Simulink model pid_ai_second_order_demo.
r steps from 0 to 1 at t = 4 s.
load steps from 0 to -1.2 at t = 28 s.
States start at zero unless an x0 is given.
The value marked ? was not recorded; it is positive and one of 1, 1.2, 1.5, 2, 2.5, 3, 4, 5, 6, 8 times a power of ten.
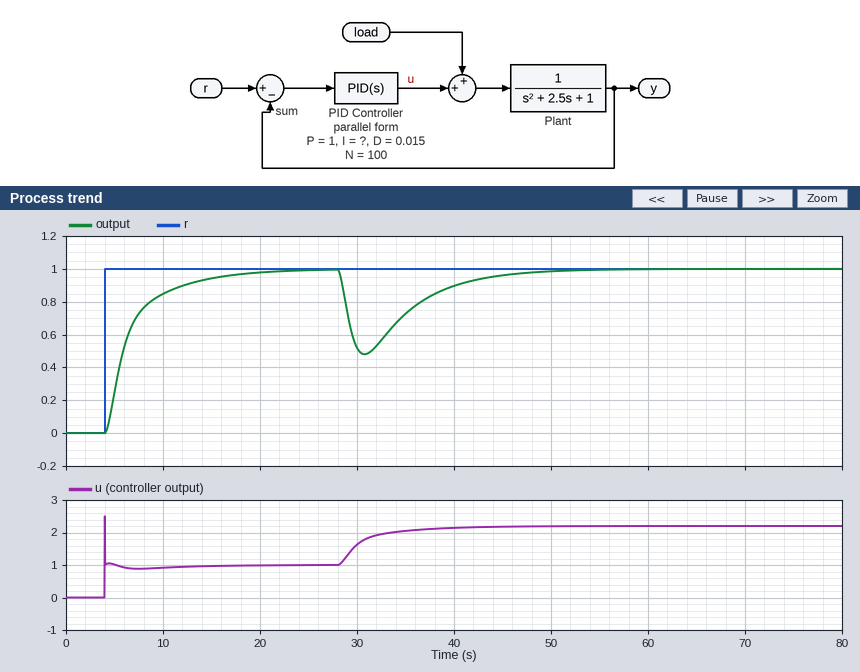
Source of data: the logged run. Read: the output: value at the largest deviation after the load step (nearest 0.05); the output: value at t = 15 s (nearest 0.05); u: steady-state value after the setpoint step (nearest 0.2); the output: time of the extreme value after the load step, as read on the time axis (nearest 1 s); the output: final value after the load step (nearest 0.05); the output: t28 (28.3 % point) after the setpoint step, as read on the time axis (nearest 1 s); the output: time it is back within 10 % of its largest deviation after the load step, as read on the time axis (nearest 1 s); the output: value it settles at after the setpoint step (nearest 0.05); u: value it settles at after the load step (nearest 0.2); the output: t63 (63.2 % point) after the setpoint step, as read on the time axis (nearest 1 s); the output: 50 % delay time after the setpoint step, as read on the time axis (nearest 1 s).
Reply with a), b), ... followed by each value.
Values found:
a) 0.50
b) 0.95
c) 1.0
d) 31 s
e) 1.00
f) 5 s
g) 44 s
h) 1.00
i) 2.2
j) 7 s
k) 6 s
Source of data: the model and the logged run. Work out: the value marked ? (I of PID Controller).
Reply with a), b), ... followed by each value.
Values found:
a) 0.3
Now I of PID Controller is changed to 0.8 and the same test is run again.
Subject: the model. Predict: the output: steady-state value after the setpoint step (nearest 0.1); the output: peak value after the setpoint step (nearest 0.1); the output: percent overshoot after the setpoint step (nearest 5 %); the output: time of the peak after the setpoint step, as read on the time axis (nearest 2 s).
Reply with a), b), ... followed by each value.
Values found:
a) 1.0
b) 1.1
c) 10 %
d) 8 s
